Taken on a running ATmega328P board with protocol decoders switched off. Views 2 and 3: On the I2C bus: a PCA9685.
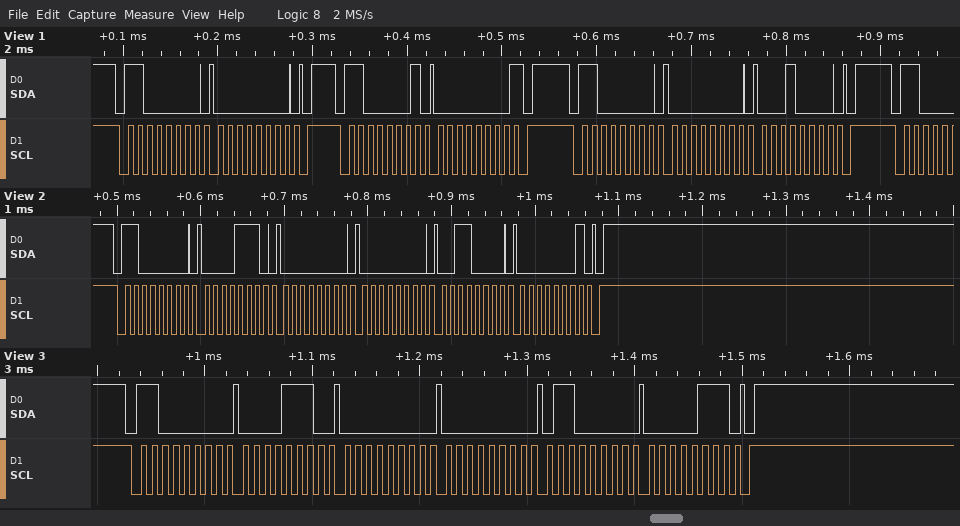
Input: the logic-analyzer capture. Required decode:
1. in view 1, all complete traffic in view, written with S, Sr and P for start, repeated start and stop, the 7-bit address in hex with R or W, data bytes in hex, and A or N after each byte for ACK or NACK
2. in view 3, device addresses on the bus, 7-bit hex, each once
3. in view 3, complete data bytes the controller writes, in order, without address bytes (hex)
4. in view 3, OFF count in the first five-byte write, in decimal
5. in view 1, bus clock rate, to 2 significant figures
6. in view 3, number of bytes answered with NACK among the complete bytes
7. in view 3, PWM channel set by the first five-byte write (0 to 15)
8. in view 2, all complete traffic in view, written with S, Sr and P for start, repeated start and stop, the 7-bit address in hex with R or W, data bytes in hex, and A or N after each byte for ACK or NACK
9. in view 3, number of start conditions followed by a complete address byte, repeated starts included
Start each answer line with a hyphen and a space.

- S 60W A 00 A P S 60R A 00 N P S 60W A 00 A 10 A P
- 0x60
- 0E 00 00 60 07
- 1888
- 100 kHz
- 0
- 2
- S 60W A 0E A 00 A 00 A 30 A 01 A P
- 1
